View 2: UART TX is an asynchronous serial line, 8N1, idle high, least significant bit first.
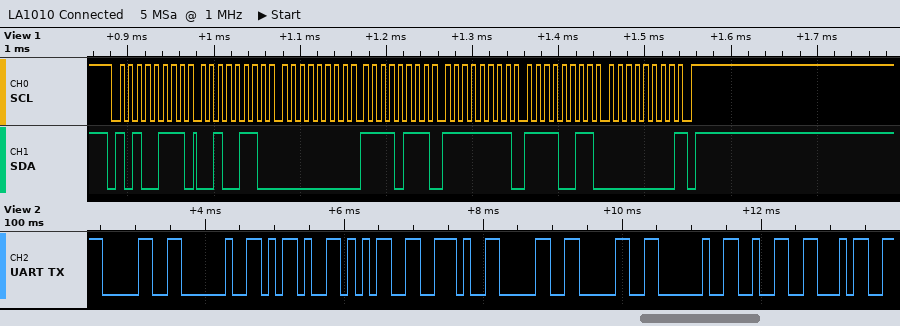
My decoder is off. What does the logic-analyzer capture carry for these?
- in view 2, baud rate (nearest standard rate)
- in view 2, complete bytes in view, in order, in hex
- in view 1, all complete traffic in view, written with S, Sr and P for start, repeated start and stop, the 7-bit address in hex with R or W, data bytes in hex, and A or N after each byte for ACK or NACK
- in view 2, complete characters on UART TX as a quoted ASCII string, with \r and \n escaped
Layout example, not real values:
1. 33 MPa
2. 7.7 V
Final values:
1. 9600 baud
2. 30 20 2D 35 2E 30 30 20 32 34
3. S 53R A 26 A 00 A F7 A FF A F3 A 00 N P
4. "0 -5.00 24"
